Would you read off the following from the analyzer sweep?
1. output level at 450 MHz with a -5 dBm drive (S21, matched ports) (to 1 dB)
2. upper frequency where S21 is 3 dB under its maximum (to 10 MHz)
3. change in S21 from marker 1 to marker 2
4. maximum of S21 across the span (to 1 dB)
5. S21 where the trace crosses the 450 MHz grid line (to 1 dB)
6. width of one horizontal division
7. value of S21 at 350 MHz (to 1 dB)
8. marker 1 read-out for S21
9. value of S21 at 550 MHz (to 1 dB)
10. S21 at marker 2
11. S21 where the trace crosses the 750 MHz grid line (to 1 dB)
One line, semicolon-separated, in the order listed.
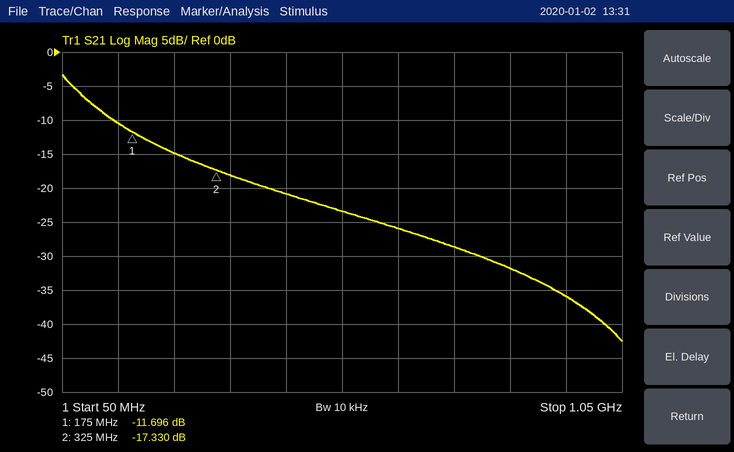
-26 dBm; 90 MHz; -5.634 dB; -3 dB; -21 dB; 100 MHz; -18 dB; -11.696 dB; -23 dB; -17.330 dB; -29 dB
